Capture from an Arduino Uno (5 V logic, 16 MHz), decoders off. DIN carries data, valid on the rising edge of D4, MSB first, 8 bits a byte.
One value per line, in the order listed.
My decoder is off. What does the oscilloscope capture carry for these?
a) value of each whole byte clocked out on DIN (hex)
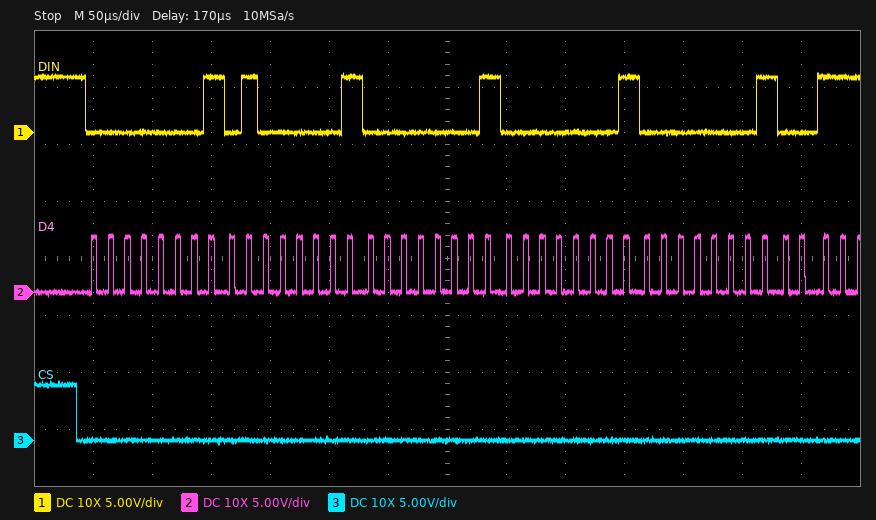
01 41 01 01 01
